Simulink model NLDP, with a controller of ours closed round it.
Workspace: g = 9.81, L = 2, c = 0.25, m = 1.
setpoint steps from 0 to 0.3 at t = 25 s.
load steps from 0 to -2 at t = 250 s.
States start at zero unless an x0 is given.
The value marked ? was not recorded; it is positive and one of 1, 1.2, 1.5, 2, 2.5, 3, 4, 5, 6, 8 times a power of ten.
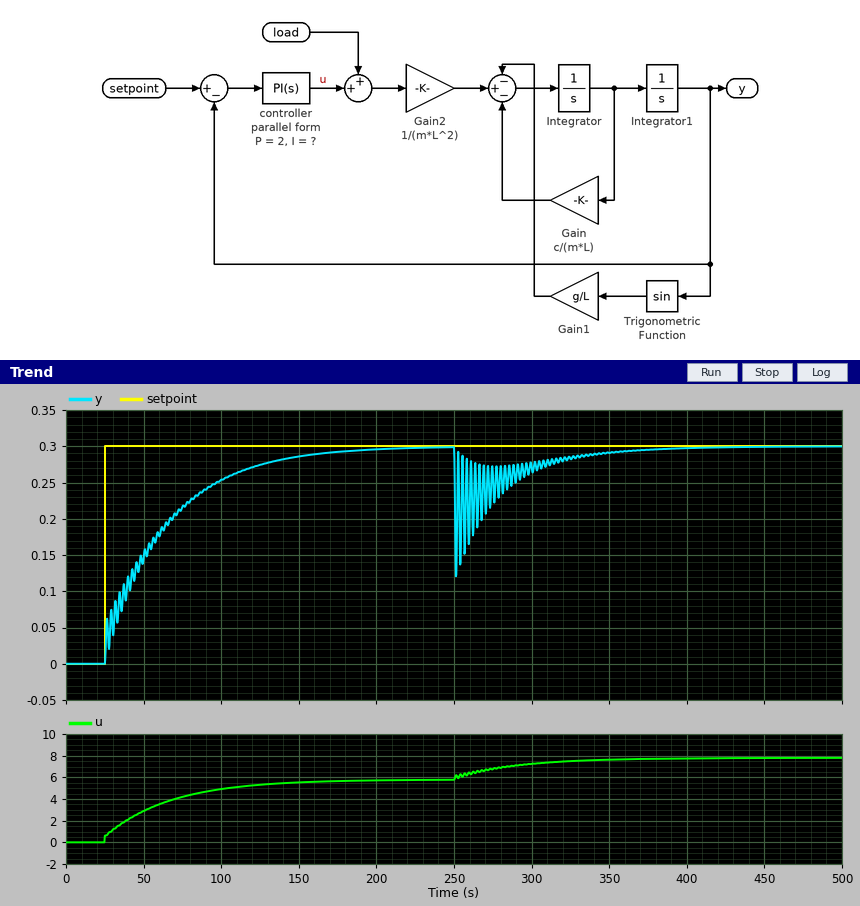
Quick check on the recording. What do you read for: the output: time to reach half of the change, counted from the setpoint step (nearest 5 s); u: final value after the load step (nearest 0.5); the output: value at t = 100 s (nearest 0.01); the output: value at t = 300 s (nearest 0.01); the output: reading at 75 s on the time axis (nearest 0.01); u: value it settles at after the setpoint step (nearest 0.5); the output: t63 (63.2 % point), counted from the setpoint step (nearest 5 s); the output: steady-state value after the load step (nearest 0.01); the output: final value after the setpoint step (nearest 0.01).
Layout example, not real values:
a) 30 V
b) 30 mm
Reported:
a) 25 s
b) 8.0
c) 0.25
d) 0.27
e) 0.22
f) 6.0
g) 40 s
h) 0.30
i) 0.30
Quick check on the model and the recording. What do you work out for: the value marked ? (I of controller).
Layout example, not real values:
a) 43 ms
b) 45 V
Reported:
a) 0.5
